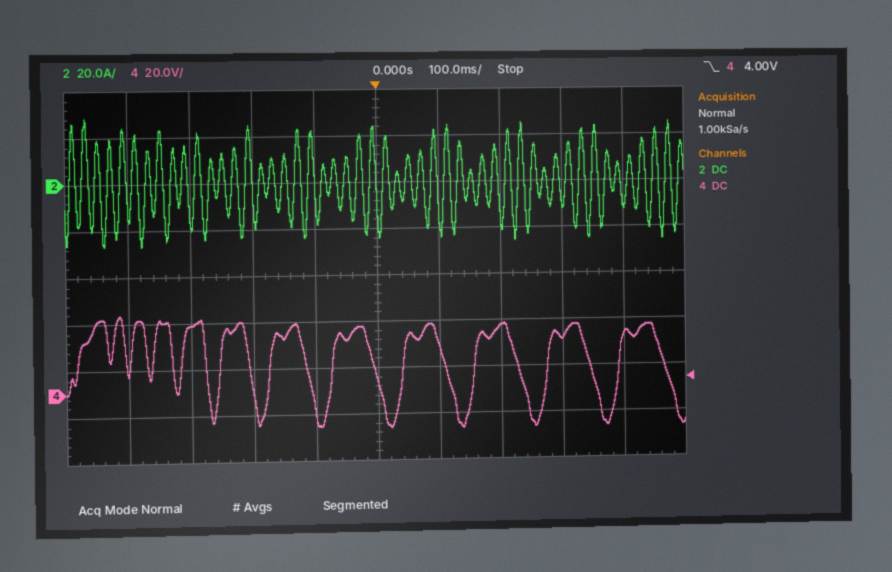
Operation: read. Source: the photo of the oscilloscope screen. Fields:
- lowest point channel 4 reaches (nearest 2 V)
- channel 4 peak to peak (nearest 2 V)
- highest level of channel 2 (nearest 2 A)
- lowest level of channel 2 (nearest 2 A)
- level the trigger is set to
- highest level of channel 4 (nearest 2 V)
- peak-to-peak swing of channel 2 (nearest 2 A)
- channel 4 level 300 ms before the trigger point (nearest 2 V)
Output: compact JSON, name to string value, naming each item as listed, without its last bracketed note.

{"lowest point channel 4 reaches": "-16 V", "channel 4 peak to peak": "50 V", "highest level of channel 2": "28 A", "lowest level of channel 2": "-26 A", "level the trigger is set to": "4.00 V", "highest level of channel 4": "34 V", "peak-to-peak swing of channel 2": "54 A", "channel 4 level 300 ms before the trigger point": "30 V"}
